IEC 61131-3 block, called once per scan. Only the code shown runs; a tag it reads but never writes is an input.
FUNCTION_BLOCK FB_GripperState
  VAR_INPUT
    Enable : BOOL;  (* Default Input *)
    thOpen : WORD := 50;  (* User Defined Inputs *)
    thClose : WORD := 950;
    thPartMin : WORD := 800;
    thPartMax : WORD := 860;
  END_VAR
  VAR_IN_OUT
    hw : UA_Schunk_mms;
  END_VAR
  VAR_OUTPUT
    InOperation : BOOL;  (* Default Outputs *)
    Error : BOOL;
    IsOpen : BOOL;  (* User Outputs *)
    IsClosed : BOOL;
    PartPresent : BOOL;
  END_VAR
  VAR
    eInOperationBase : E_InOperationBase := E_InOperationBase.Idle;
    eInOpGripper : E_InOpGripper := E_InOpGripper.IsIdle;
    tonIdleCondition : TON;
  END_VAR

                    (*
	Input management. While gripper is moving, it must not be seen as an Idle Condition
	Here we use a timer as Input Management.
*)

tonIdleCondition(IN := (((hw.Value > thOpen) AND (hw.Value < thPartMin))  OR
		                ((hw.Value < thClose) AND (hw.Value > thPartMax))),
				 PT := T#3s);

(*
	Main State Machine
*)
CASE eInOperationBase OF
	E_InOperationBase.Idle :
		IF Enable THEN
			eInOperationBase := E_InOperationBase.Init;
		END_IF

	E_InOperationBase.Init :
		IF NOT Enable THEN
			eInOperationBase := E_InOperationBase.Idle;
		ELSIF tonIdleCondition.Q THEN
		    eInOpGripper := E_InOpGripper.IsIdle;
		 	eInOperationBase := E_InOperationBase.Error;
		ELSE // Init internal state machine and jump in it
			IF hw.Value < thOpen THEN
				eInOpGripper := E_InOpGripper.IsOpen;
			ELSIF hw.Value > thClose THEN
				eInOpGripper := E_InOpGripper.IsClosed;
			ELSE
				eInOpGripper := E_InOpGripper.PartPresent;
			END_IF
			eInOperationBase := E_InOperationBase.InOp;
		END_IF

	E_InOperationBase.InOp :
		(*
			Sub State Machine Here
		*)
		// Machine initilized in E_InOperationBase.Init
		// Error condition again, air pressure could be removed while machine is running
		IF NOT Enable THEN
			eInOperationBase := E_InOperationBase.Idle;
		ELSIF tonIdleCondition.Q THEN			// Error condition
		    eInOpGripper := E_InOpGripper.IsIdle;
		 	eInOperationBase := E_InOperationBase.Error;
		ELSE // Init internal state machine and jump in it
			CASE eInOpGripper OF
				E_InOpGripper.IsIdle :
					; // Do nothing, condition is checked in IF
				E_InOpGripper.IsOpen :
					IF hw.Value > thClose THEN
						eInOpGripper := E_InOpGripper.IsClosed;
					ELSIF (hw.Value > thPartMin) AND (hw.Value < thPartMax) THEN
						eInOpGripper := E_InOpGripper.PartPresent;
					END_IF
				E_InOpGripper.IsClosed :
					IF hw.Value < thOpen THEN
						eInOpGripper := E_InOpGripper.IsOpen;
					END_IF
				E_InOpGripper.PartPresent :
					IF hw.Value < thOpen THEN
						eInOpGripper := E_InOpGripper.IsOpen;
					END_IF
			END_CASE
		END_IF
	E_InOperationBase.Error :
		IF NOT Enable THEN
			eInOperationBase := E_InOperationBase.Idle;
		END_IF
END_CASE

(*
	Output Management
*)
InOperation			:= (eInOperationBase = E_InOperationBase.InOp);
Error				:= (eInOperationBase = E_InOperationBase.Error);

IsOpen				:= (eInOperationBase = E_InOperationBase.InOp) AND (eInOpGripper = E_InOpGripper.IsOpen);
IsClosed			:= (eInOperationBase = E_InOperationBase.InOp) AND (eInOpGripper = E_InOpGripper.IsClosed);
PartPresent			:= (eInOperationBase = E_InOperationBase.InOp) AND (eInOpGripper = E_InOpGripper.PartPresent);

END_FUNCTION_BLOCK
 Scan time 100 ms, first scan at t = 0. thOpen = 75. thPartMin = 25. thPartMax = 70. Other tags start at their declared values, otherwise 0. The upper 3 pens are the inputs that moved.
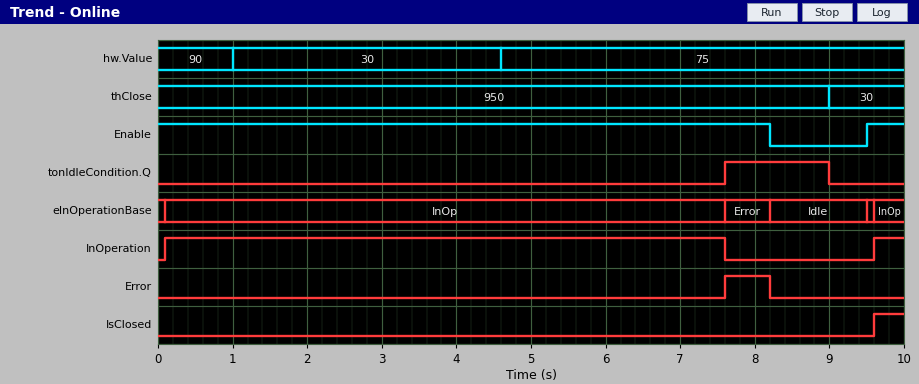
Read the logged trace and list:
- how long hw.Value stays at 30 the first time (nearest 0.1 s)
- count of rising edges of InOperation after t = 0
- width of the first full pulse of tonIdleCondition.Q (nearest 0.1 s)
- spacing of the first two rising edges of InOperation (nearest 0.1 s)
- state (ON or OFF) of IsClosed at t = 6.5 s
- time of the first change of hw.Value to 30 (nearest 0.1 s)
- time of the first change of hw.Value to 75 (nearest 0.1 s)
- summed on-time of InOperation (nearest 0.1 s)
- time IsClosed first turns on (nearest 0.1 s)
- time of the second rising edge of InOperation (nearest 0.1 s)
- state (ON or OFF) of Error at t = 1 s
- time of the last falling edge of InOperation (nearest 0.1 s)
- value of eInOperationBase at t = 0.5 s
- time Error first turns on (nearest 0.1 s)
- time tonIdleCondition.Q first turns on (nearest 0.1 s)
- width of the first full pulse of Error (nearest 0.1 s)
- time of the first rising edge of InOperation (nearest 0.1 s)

3.6 s
2
1.4 s
9.5 s
OFF
1.0 s
4.6 s
7.9 s
9.6 s
9.6 s
OFF
7.6 s
InOp
7.6 s
7.6 s
0.6 s
0.1 s
